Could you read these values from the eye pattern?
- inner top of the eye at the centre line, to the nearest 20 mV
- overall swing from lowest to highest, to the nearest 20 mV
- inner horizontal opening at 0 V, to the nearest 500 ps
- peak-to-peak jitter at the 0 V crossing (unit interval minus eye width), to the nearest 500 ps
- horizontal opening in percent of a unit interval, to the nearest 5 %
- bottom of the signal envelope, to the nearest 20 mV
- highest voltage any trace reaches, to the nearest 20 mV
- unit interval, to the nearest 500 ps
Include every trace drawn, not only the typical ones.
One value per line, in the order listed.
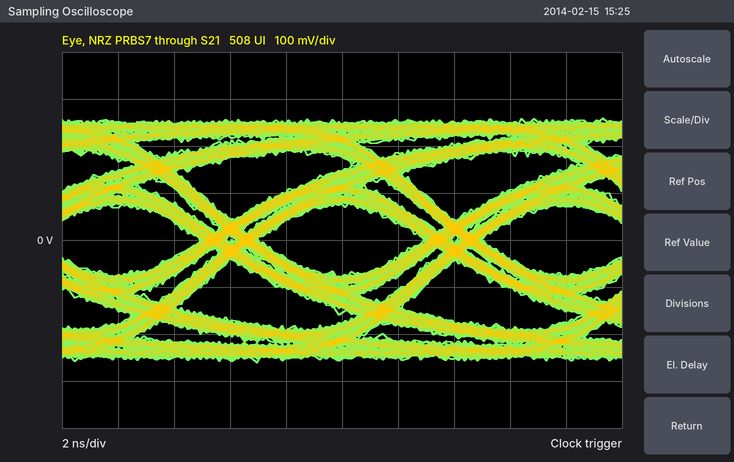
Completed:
80 mV
520 mV
6.0 ns
2.0 ns
75 %
-260 mV
260 mV
8.0 ns
